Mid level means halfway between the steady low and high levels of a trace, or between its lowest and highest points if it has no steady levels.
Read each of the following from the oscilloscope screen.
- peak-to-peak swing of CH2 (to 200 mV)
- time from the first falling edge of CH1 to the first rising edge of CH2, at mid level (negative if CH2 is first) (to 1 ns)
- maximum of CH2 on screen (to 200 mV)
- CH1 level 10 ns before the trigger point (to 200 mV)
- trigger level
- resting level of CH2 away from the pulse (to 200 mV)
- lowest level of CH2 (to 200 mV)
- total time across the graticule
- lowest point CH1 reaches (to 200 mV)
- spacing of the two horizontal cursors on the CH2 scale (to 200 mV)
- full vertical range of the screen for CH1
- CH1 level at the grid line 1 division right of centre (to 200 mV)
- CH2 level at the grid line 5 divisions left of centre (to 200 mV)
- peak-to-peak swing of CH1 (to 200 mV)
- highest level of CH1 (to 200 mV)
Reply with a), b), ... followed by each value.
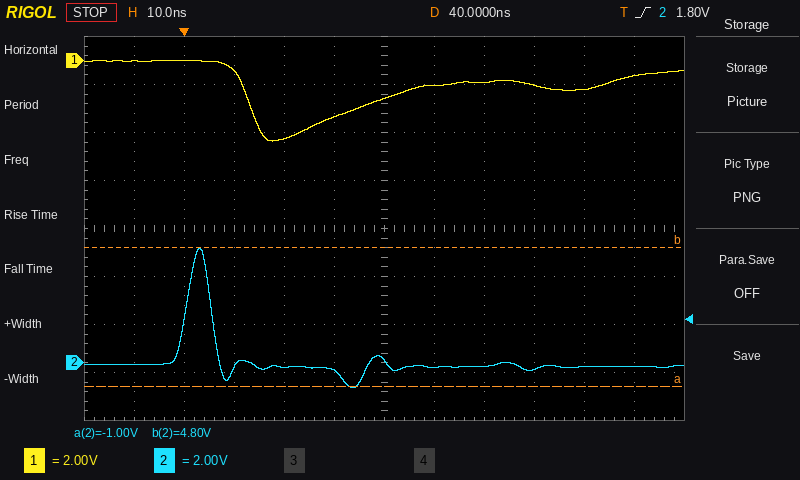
a) 5.8 V
b) -13 ns
c) 4.8 V
d) 0.0 V
e) 1.80 V
f) -200 mV
g) -1.0 V
h) 120 ns
i) -3.4 V
j) 5.8 V
k) 16 V
l) -1.0 V
m) 0.0 V
n) 3.4 V
o) 0.0 V
